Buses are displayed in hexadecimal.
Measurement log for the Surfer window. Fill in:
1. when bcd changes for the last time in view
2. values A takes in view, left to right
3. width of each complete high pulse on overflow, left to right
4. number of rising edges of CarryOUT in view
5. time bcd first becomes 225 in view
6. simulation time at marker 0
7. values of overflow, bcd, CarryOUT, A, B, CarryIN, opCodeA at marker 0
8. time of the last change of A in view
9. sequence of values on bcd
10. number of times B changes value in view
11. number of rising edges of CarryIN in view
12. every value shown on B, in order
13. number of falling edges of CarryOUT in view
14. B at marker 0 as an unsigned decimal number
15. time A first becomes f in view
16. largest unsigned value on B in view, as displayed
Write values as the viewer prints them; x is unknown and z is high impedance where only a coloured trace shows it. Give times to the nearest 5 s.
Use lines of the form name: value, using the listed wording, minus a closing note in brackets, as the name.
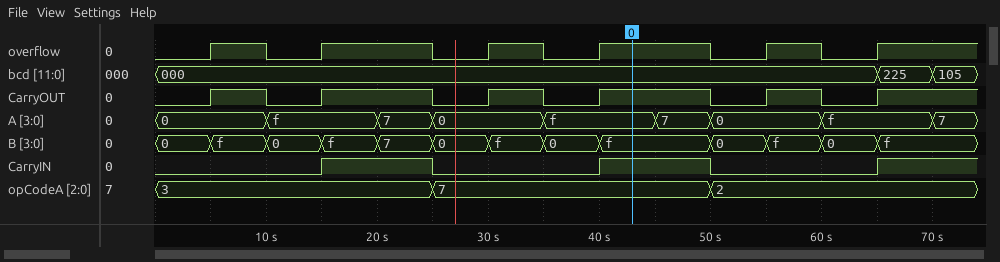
when bcd changes for the last time in view: 70 s
values A takes in view, left to right: 0, f, 7, 0, f, 7, 0, f, 7
width of each complete high pulse on overflow, left to right: 5 s, 10 s, 5 s, 10 s, 5 s
number of rising edges of CarryOUT in view: 6
time bcd first becomes 225 in view: 65 s
simulation time at marker 0: 45 s
values of overflow, bcd, CarryOUT, A, B, CarryIN, opCodeA at marker 0: overflow=1, bcd=000, CarryOUT=1, A=f, B=f, CarryIN=1, opCodeA=7
time of the last change of A in view: 70 s
sequence of values on bcd: 000, 225, 105
number of times B changes value in view: 12
number of rising edges of CarryIN in view: 3
every value shown on B, in order: 0, f, 0, f, 7, 0, f, 0, f, 0, f, 0, f
number of falling edges of CarryOUT in view: 5
B at marker 0 as an unsigned decimal number: 15
time A first becomes f in view: 10 s
largest unsigned value on B in view, as displayed: f
